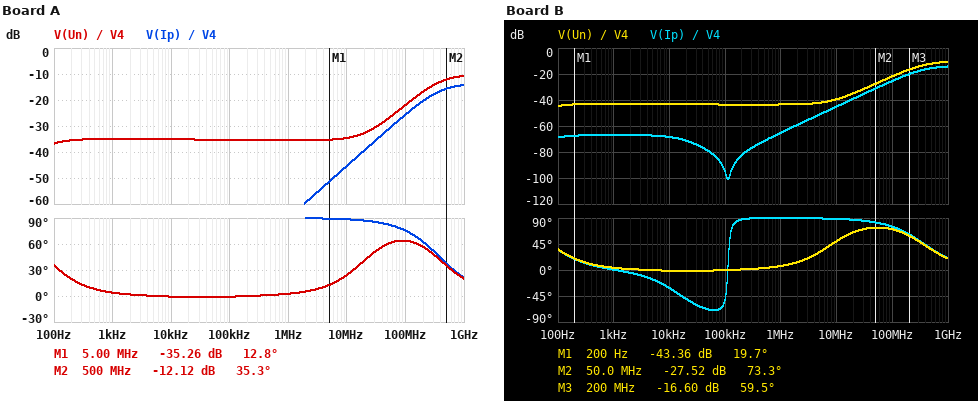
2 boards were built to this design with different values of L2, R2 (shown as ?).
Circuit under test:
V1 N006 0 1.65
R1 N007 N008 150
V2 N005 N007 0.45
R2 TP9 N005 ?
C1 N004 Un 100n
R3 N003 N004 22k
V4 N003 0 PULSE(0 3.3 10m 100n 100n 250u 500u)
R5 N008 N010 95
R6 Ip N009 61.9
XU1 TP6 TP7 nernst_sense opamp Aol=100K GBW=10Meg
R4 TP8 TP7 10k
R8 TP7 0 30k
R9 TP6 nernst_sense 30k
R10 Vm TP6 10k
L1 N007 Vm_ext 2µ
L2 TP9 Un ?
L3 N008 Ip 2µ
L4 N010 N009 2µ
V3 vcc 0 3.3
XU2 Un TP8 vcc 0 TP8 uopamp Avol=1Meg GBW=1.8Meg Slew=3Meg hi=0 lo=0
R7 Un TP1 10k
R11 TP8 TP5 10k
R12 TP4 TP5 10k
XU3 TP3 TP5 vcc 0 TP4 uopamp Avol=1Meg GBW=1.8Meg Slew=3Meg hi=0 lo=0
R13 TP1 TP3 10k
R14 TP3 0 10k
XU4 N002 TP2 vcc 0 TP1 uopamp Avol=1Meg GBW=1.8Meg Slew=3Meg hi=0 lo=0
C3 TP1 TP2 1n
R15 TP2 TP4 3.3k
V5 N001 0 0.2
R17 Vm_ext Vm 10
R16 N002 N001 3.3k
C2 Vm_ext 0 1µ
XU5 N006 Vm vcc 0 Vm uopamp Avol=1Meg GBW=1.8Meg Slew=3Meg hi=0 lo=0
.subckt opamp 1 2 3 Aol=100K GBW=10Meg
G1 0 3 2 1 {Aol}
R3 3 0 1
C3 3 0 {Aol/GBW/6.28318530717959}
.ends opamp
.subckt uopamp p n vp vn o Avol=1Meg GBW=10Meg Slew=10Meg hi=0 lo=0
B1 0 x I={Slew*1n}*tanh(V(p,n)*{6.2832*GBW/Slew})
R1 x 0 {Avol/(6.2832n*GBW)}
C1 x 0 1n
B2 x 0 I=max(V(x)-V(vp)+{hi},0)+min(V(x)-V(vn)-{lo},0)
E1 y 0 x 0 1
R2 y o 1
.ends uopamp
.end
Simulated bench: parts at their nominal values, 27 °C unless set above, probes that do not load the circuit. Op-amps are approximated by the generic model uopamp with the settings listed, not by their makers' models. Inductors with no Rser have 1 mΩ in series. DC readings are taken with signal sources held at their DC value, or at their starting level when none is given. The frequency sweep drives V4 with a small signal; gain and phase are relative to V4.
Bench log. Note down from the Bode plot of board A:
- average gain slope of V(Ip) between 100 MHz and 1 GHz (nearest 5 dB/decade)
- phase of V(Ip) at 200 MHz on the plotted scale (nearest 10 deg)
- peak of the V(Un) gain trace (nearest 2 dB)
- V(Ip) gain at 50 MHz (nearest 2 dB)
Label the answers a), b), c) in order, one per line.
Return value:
a) 10 dB/decade
b) 60 deg
c) -10 dB
d) -32 dB
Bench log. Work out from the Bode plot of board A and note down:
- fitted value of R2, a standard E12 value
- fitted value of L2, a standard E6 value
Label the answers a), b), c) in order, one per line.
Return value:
a) 390 Ω
b) 1 µH
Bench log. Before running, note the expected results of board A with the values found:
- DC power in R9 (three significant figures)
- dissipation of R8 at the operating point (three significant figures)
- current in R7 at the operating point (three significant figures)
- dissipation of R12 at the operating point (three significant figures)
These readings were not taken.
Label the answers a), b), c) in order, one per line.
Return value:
a) 1.43 µW
b) 83.3 µW
c) 20.0 µA
d) 91.0 µW
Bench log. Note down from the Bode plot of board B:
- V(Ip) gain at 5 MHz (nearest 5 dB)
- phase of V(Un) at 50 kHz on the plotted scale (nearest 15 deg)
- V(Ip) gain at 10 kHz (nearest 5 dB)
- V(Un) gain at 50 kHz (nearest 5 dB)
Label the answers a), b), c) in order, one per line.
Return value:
a) -50 dB
b) 0 deg
c) -70 dB
d) -45 dB
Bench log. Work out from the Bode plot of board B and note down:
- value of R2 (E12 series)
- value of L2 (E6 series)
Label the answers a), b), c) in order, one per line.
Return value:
a) 150 Ω
b) 1 µH
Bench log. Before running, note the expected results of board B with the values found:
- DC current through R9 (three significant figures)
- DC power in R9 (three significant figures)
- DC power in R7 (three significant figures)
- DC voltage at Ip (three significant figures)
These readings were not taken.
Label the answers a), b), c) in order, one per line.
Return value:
a) 7.26 µA
b) 1.58 µW
c) 4.00 µW
d) 1.65 V
